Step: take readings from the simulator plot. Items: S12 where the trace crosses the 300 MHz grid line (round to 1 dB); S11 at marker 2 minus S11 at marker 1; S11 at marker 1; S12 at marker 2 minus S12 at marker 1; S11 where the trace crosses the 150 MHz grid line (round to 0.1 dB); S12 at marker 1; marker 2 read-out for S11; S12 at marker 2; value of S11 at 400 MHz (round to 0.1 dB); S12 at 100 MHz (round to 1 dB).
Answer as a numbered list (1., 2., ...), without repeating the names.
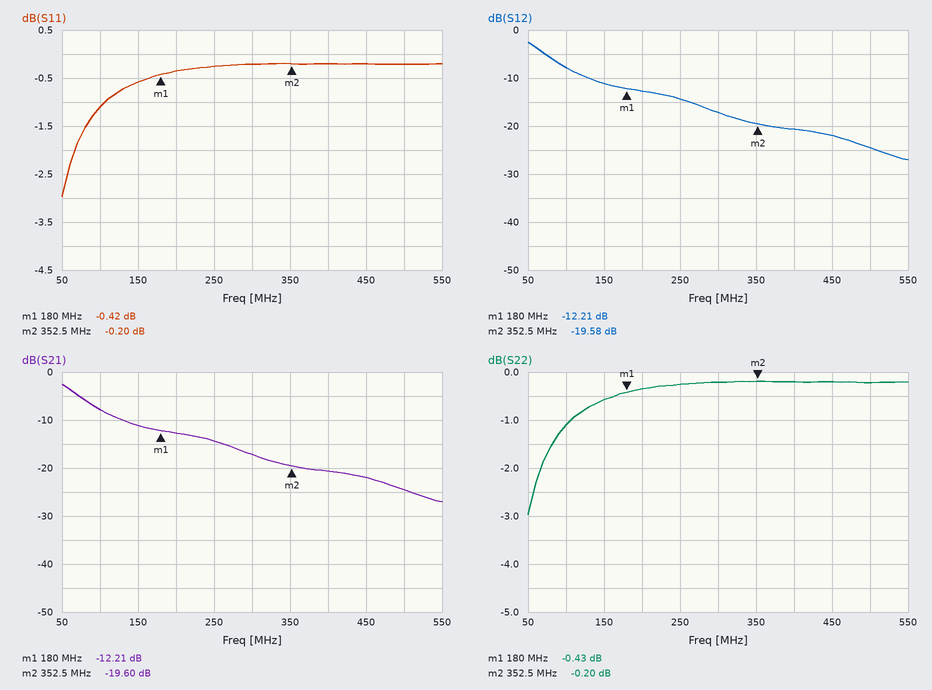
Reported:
1. -17 dB
2. 0.22 dB
3. -0.42 dB
4. -7.37 dB
5. -0.6 dB
6. -12.21 dB
7. -0.20 dB
8. -19.58 dB
9. -0.2 dB
10. -8 dB
